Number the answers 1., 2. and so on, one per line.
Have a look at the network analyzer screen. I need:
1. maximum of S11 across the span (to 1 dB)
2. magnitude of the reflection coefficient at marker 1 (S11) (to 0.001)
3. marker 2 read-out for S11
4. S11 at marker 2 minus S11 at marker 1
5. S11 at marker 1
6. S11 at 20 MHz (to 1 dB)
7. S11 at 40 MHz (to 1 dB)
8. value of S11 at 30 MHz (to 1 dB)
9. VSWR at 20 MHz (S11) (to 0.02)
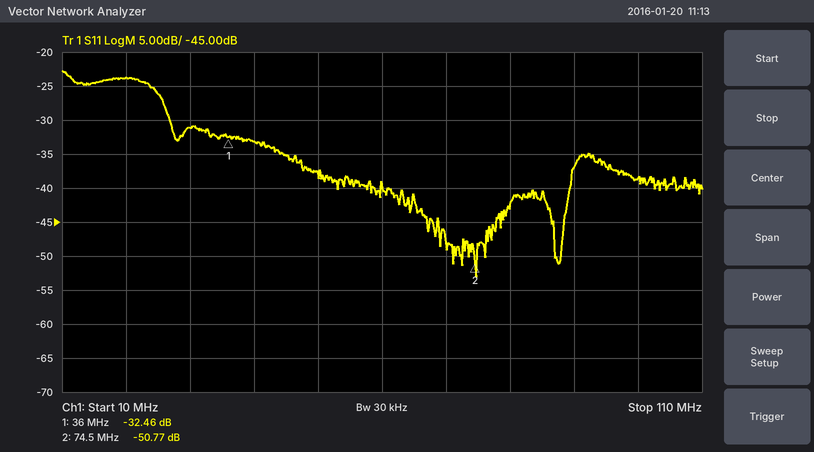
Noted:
1. -23 dB
2. 0.024
3. -50.77 dB
4. -18.31 dB
5. -32.46 dB
6. -24 dB
7. -33 dB
8. -31 dB
9. 1.14
